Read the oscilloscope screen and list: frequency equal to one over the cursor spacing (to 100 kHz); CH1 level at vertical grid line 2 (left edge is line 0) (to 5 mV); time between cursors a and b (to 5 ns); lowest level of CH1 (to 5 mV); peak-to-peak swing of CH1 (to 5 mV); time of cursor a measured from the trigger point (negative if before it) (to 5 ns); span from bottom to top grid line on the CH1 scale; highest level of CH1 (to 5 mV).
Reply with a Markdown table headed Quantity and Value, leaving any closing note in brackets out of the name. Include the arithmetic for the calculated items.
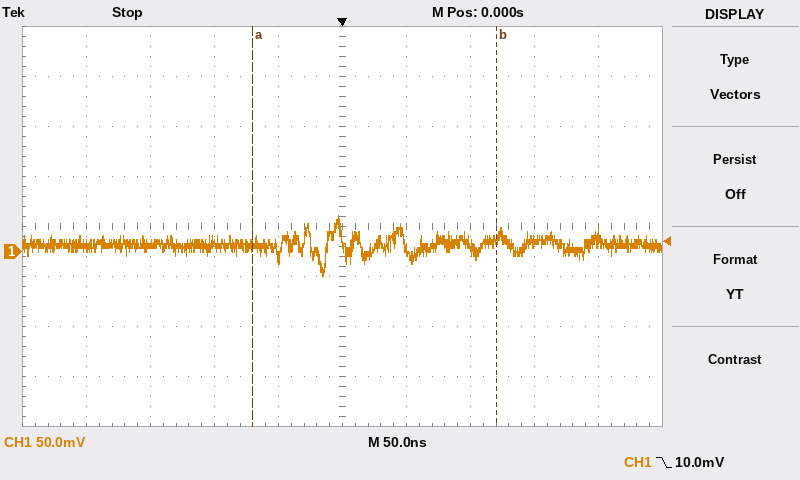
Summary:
| Quantity | Value |
|---|---|
| frequency equal to one over the cursor spacing | 1 / 190 ns ≈ 5.3 MHz |
| CH1 level at vertical grid line 2 (left edge is line 0) | 10 mV |
| time between cursors a and b | 190 ns |
| lowest level of CH1 | -25 mV |
| peak-to-peak swing of CH1 | 35 mV − (-25 mV) = 60 mV |
| time of cursor a measured from the trigger point (negative if before it) | -70 ns |
| span from bottom to top grid line on the CH1 scale | 400 mV |
| highest level of CH1 | 35 mV |
